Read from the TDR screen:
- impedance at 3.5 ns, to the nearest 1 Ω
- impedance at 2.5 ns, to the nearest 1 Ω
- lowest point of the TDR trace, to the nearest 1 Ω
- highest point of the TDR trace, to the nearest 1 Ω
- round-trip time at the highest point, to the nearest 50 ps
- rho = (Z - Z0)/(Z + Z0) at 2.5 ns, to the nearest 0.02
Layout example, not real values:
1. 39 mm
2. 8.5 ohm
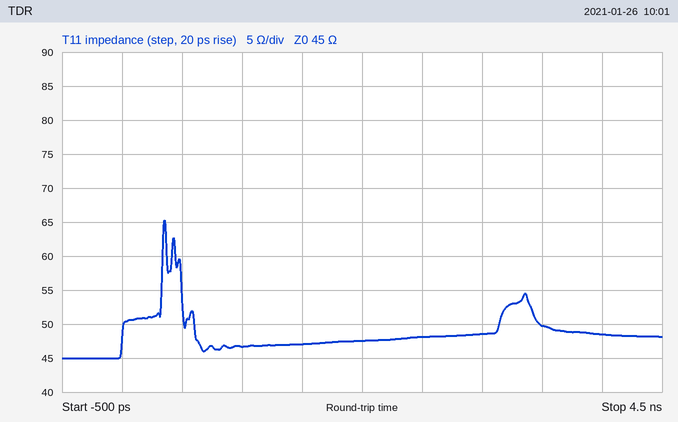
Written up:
1. 50 Ω
2. 48 Ω
3. 45 Ω
4. 65 Ω
5. 350 ps
6. +0.04
